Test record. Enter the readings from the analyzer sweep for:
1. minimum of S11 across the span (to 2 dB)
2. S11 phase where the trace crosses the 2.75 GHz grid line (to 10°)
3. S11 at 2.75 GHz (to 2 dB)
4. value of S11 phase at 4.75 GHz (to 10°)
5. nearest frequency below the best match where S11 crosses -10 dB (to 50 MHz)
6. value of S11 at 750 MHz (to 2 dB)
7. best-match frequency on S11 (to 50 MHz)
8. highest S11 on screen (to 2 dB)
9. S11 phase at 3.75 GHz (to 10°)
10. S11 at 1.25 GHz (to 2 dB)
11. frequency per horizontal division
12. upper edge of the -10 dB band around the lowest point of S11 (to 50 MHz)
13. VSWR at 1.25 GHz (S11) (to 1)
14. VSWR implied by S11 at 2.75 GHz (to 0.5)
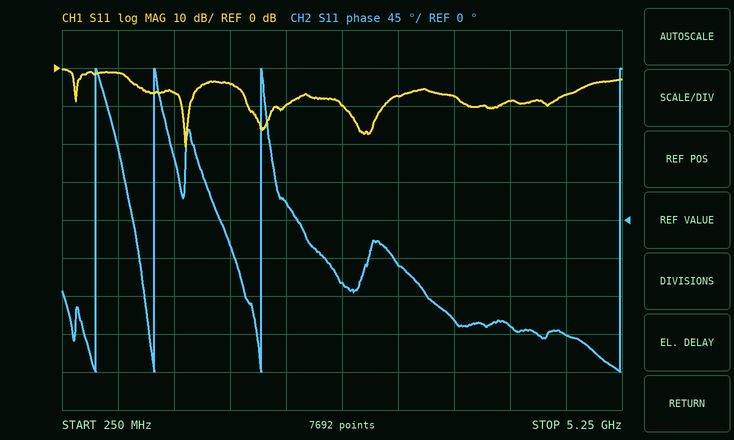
-20 dB
-70°
-10 dB
-140°
1.30 GHz
-2 dB
1.35 GHz
0 dB
-120°
-6 dB
500 MHz
1.40 GHz
3
2.0
